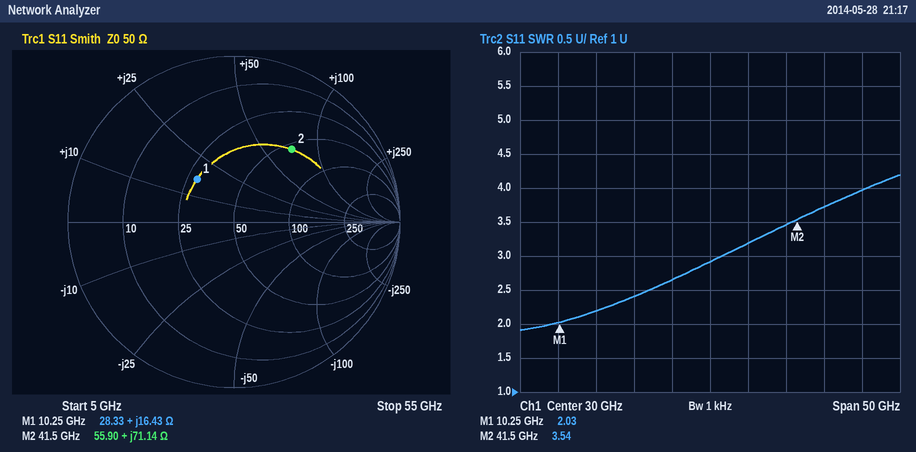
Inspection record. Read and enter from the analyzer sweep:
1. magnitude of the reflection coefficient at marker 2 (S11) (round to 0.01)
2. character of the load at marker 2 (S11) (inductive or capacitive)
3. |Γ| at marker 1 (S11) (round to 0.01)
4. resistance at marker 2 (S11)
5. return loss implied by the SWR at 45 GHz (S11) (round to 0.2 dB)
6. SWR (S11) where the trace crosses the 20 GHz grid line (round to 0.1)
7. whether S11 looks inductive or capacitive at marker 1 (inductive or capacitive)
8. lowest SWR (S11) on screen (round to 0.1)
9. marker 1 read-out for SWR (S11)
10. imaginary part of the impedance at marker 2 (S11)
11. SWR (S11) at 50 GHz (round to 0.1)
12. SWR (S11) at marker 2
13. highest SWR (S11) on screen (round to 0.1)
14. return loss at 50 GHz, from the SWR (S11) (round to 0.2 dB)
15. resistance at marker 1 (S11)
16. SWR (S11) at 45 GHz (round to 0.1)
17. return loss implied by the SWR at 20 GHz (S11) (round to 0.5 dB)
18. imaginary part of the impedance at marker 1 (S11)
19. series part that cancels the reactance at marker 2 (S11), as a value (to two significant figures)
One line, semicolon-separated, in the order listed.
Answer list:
0.56; inductive; 0.34; 55.90 Ω; 4.8 dB; 2.4; inductive; 1.9; 2.03; +71.14 Ω; 4.0; 3.54; 4.2; 4.4 dB; 28.33 Ω; 3.7; 7.5 dB; +16.43 Ω; 54 fF
